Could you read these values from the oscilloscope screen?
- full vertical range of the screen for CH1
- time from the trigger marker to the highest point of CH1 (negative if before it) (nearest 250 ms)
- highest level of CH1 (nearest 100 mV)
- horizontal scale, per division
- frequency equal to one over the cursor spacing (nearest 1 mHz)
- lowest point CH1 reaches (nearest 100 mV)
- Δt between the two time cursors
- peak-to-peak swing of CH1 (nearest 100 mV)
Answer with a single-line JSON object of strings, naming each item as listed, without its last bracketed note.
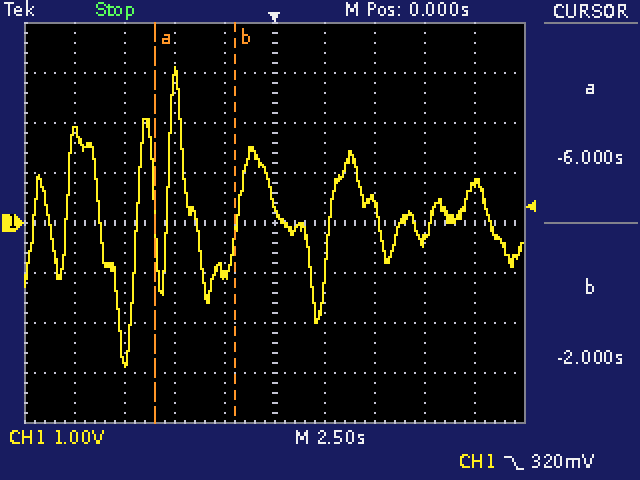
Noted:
{"full vertical range of the screen for CH1": "8 V", "time from the trigger marker to the highest point of CH1 (negative if before it)": "-5.00 s", "highest level of CH1": "3.1 V", "horizontal scale, per division": "2.5 s", "frequency equal to one over the cursor spacing": "250 mHz", "lowest point CH1 reaches": "-2.9 V", "Δt between the two time cursors": "4.00 s", "peak-to-peak swing of CH1": "6.0 V"}
